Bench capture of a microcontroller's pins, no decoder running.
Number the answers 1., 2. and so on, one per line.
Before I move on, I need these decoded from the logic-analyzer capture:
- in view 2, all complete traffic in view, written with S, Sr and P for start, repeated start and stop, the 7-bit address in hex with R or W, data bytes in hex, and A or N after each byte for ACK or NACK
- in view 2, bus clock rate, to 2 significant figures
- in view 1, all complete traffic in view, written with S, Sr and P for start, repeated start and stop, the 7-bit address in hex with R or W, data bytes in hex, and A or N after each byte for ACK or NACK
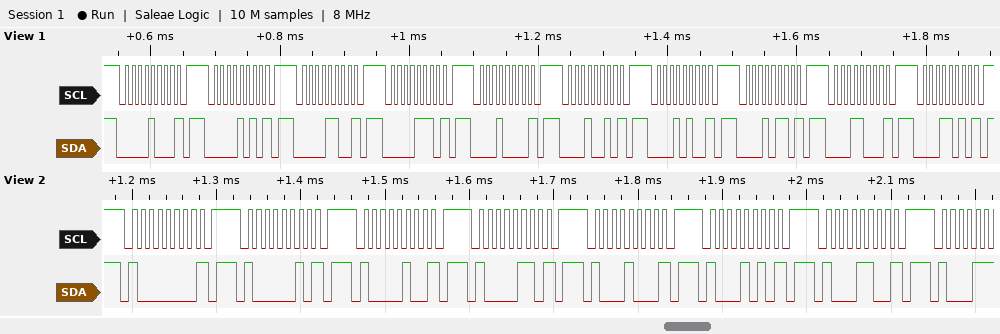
1. S 40W N P S 41W N P S 42W N P S 43W N P S 44W N P S 45W N P S 46W N P
2. 100 kHz
3. S 04W N P S 05W N P S 06W N P S 07W N P S 08W N P S 09W N P S 0AW N P S 0BW N P S 0CW N P S 0DW N P
